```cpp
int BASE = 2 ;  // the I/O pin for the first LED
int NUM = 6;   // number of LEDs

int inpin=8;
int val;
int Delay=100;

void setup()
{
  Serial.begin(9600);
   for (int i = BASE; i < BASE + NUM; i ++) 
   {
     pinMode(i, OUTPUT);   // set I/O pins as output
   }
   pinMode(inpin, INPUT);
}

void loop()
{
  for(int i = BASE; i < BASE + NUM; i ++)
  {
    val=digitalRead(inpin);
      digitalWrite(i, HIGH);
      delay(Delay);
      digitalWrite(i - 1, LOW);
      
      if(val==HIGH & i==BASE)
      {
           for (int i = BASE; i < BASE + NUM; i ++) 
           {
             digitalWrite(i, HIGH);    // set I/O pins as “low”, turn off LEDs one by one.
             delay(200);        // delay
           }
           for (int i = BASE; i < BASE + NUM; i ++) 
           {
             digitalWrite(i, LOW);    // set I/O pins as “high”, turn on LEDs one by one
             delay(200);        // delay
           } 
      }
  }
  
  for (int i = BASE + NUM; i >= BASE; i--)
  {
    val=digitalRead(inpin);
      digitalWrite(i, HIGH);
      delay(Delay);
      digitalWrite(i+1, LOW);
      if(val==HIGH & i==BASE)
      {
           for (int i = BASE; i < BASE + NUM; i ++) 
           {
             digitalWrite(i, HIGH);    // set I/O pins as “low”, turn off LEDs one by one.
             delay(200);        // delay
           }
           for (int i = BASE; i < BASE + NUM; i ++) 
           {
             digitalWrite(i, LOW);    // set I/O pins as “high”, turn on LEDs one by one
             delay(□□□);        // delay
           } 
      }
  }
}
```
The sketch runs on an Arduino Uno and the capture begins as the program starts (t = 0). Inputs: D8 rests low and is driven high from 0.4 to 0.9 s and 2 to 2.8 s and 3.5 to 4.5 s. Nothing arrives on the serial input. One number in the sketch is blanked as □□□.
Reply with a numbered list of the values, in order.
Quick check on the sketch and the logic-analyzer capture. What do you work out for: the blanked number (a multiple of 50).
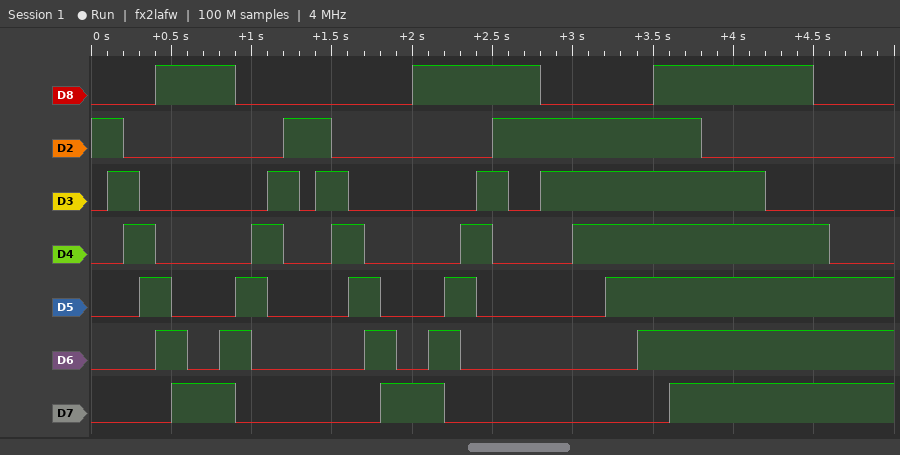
1. 400
